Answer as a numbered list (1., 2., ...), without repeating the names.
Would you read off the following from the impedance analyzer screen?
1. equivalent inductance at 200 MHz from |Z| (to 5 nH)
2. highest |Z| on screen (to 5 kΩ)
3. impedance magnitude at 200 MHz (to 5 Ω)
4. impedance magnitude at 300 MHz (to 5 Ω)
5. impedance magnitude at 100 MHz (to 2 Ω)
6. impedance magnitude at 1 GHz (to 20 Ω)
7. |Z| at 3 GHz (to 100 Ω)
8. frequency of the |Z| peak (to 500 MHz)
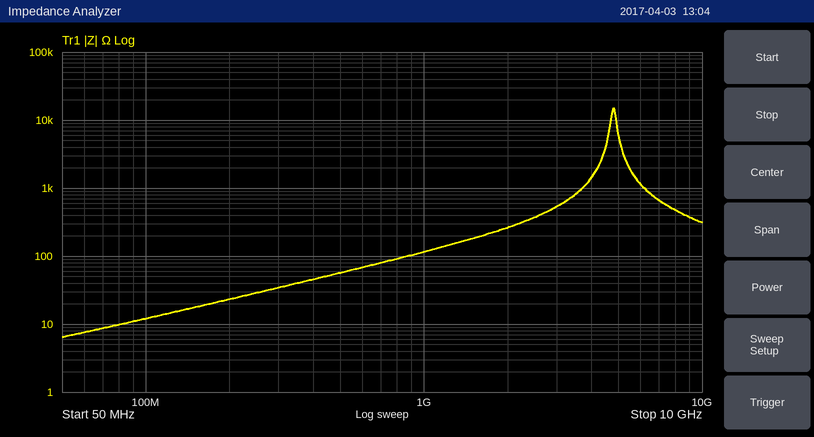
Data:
1. 20 nH
2. 15 kΩ
3. 25 Ω
4. 35 Ω
5. 12 Ω
6. 120 Ω
7. 500 Ω
8. 5.0 GHz
